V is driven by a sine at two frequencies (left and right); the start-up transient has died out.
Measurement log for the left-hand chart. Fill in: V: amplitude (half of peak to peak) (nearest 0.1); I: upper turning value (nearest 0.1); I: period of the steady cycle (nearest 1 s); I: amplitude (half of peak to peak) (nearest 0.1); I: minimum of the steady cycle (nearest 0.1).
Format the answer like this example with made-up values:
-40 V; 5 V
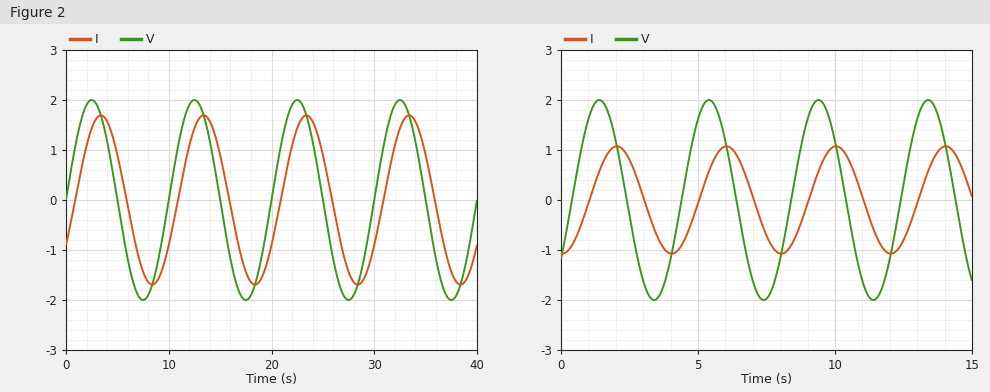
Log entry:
2.0; 1.7; 10 s; 1.7; -1.7
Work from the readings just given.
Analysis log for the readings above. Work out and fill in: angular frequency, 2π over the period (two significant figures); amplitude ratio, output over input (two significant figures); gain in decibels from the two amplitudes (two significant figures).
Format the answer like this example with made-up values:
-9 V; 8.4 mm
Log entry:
0.63 rad/s; 0.85; -1.4 dB
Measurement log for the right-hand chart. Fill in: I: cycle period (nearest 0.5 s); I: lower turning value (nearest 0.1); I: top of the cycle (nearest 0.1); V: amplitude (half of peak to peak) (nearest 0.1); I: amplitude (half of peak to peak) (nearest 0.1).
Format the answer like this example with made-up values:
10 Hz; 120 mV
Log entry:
4.0 s; -1.1; 1.1; 2.0; 1.1
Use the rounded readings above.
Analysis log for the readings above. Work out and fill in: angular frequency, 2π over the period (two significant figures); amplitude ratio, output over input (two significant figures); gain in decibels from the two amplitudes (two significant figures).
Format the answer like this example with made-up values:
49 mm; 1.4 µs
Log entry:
1.6 rad/s; 0.55; -5.2 dB
